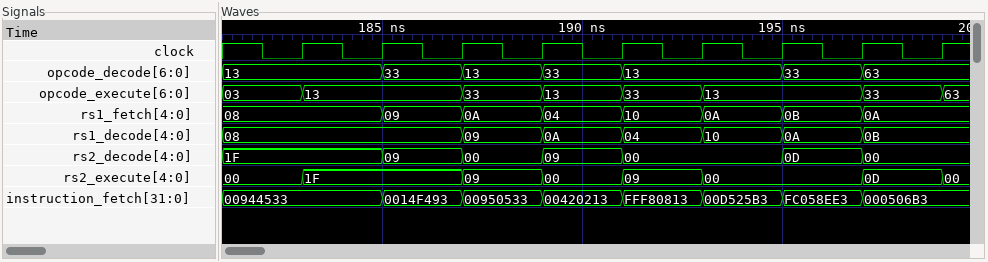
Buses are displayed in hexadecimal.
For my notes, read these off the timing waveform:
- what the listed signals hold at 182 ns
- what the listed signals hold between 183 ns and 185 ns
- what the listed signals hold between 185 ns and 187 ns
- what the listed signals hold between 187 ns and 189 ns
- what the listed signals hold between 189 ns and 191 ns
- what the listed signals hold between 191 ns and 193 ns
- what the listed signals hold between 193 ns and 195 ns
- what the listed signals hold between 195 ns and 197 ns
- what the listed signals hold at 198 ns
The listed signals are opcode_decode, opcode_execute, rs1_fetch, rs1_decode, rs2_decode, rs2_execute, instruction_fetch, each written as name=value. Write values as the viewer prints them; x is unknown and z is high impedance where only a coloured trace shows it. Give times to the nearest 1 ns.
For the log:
opcode_decode=13, opcode_execute=03, rs1_fetch=08, rs1_decode=08, rs2_decode=1F, rs2_execute=00, instruction_fetch=00944533
opcode_decode=13, opcode_execute=13, rs1_fetch=08, rs1_decode=08, rs2_decode=1F, rs2_execute=1F, instruction_fetch=00944533
opcode_decode=33, opcode_execute=13, rs1_fetch=09, rs1_decode=08, rs2_decode=09, rs2_execute=1F, instruction_fetch=0014F493
opcode_decode=13, opcode_execute=33, rs1_fetch=0A, rs1_decode=09, rs2_decode=00, rs2_execute=09, instruction_fetch=00950533
opcode_decode=33, opcode_execute=13, rs1_fetch=04, rs1_decode=0A, rs2_decode=09, rs2_execute=00, instruction_fetch=00420213
opcode_decode=13, opcode_execute=33, rs1_fetch=10, rs1_decode=04, rs2_decode=00, rs2_execute=09, instruction_fetch=FFF80813
opcode_decode=13, opcode_execute=13, rs1_fetch=0A, rs1_decode=10, rs2_decode=00, rs2_execute=00, instruction_fetch=00D525B3
opcode_decode=33, opcode_execute=13, rs1_fetch=0B, rs1_decode=0A, rs2_decode=0D, rs2_execute=00, instruction_fetch=FC058EE3
opcode_decode=63, opcode_execute=33, rs1_fetch=0A, rs1_decode=0B, rs2_decode=00, rs2_execute=0D, instruction_fetch=000506B3
